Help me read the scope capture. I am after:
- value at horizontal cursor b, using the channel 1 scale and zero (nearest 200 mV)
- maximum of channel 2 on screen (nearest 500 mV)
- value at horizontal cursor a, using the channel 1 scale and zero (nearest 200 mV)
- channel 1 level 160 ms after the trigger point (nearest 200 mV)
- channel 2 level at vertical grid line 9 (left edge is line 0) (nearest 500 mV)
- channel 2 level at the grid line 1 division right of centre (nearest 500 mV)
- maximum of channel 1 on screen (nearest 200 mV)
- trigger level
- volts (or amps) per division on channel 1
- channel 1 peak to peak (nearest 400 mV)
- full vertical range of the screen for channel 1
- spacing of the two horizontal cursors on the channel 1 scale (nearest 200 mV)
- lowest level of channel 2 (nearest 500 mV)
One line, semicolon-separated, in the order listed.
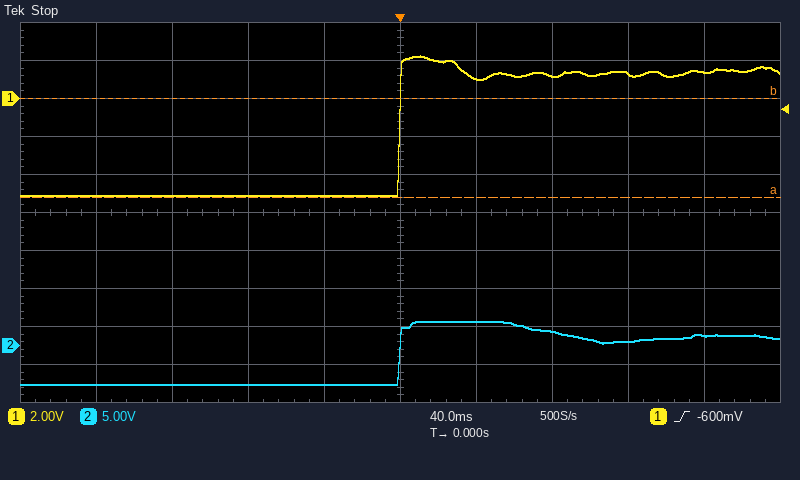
0.0 V; 3.0 V; -5.2 V; 1.4 V; 1.5 V; 3.0 V; 2.2 V; -600 mV; 2 V; 7.2 V; 20 V; 5.2 V; -5.0 V
